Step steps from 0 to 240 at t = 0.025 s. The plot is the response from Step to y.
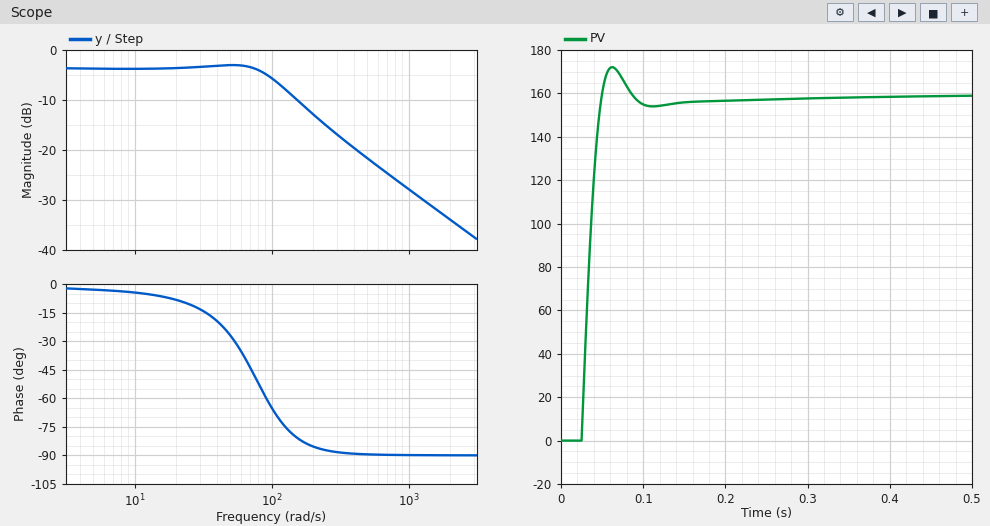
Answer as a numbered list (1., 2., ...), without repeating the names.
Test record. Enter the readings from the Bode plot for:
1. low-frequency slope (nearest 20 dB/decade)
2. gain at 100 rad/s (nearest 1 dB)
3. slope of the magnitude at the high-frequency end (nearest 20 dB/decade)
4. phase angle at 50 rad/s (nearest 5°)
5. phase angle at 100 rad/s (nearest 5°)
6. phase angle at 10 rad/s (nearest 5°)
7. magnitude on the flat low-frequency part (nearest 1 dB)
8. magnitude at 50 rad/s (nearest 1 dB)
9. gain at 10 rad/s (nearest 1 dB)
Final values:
1. 0 dB/decade
2. -6 dB
3. -20 dB/decade
4. -25°
5. -65°
6. -5°
7. -4 dB
8. -3 dB
9. -4 dB
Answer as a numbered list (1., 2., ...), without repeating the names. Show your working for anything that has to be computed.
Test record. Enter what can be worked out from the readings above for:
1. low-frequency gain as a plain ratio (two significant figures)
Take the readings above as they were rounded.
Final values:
1. 10^(-4 / 20) = 0.63
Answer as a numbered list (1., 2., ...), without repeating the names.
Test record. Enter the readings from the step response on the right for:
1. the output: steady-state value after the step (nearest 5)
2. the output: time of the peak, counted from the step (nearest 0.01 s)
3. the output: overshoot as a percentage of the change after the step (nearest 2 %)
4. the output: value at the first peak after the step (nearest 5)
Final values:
1. 160
2. 0.04 s
3. 8 %
4. 170
